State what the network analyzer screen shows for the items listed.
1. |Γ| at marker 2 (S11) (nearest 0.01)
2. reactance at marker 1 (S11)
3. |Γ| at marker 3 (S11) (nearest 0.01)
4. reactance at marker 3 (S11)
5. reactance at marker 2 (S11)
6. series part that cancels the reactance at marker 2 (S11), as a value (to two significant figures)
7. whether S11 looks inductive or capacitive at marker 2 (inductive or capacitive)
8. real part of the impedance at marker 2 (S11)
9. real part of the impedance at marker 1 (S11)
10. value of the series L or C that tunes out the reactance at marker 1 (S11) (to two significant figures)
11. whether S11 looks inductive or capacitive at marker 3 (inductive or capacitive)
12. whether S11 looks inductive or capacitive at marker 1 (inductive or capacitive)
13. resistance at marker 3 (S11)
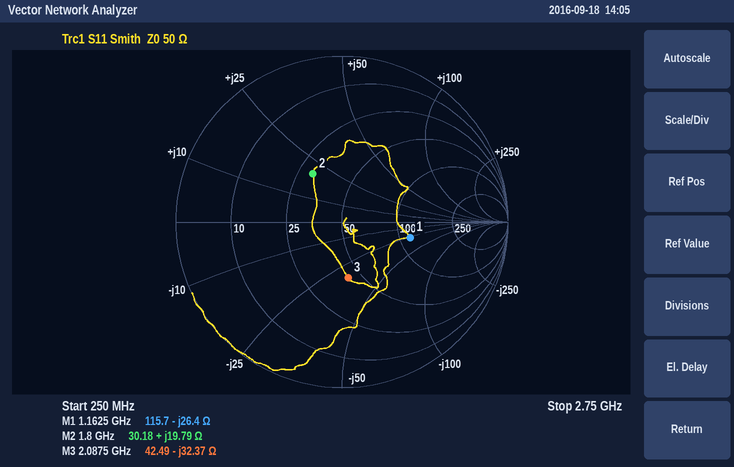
0.34
-26.4 Ω
0.34
-32.37 Ω
+19.79 Ω
4.5 pF
inductive
30.18 Ω
115.7 Ω
3.6 nH
capacitive
capacitive
42.49 Ω
